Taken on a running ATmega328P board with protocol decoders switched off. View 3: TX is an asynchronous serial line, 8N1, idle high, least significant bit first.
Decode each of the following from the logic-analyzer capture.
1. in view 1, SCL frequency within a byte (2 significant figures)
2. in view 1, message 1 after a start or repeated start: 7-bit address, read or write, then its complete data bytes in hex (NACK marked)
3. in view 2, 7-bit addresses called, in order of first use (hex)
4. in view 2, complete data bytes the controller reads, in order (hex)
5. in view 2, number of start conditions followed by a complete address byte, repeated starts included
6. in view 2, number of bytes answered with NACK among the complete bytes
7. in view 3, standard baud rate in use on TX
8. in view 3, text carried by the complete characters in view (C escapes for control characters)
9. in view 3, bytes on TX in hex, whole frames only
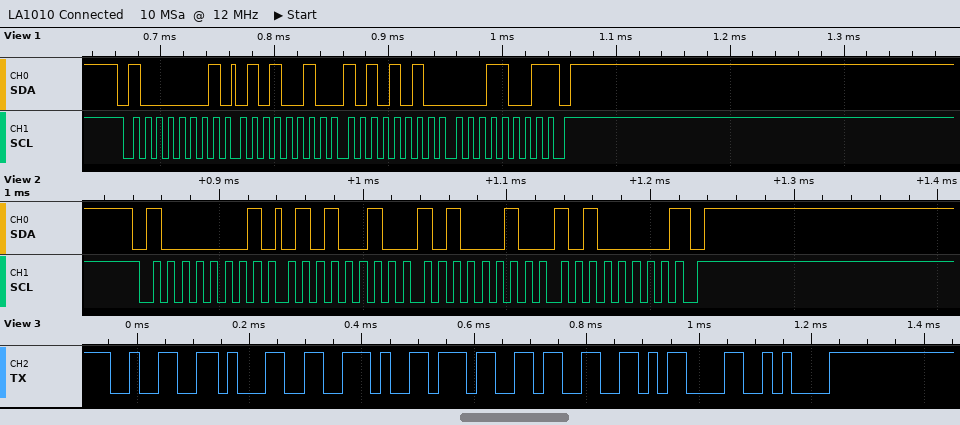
100 kHz
0x40 read: 52 AA 19 NACK
0x40
52 A2 A0
1
1
57600 baud
"21.73\r\n"
0x32 0x31 0x2E 0x37 0x33 0x0D 0x0A
